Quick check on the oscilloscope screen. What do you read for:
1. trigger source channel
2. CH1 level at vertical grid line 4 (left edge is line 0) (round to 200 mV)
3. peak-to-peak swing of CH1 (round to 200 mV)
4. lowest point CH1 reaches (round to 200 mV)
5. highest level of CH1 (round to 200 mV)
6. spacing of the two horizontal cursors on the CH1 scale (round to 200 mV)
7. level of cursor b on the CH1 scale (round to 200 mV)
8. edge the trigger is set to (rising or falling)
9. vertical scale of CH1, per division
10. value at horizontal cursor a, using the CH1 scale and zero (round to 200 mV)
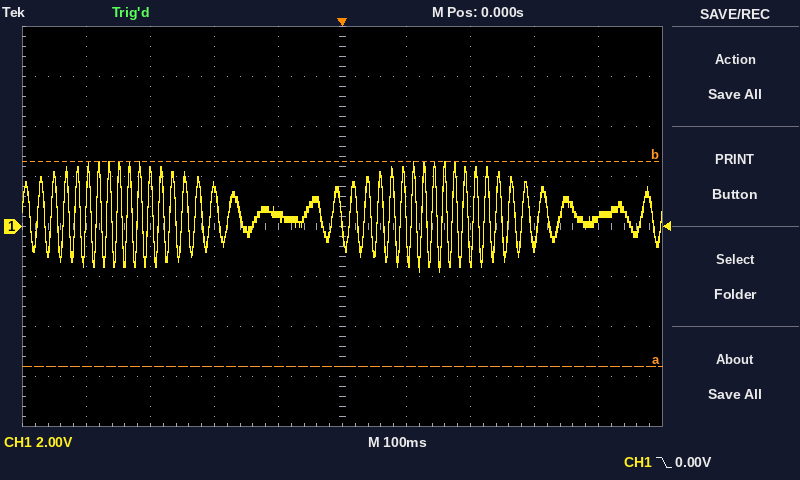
CH1
400 mV
4.4 V
-1.8 V
2.6 V
8.2 V
2.6 V
falling
2 V
-5.6 V
